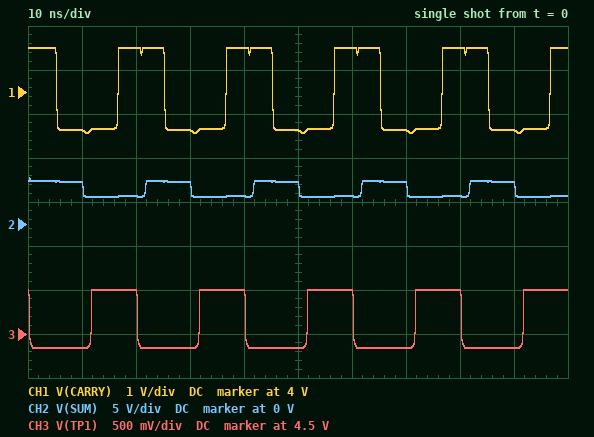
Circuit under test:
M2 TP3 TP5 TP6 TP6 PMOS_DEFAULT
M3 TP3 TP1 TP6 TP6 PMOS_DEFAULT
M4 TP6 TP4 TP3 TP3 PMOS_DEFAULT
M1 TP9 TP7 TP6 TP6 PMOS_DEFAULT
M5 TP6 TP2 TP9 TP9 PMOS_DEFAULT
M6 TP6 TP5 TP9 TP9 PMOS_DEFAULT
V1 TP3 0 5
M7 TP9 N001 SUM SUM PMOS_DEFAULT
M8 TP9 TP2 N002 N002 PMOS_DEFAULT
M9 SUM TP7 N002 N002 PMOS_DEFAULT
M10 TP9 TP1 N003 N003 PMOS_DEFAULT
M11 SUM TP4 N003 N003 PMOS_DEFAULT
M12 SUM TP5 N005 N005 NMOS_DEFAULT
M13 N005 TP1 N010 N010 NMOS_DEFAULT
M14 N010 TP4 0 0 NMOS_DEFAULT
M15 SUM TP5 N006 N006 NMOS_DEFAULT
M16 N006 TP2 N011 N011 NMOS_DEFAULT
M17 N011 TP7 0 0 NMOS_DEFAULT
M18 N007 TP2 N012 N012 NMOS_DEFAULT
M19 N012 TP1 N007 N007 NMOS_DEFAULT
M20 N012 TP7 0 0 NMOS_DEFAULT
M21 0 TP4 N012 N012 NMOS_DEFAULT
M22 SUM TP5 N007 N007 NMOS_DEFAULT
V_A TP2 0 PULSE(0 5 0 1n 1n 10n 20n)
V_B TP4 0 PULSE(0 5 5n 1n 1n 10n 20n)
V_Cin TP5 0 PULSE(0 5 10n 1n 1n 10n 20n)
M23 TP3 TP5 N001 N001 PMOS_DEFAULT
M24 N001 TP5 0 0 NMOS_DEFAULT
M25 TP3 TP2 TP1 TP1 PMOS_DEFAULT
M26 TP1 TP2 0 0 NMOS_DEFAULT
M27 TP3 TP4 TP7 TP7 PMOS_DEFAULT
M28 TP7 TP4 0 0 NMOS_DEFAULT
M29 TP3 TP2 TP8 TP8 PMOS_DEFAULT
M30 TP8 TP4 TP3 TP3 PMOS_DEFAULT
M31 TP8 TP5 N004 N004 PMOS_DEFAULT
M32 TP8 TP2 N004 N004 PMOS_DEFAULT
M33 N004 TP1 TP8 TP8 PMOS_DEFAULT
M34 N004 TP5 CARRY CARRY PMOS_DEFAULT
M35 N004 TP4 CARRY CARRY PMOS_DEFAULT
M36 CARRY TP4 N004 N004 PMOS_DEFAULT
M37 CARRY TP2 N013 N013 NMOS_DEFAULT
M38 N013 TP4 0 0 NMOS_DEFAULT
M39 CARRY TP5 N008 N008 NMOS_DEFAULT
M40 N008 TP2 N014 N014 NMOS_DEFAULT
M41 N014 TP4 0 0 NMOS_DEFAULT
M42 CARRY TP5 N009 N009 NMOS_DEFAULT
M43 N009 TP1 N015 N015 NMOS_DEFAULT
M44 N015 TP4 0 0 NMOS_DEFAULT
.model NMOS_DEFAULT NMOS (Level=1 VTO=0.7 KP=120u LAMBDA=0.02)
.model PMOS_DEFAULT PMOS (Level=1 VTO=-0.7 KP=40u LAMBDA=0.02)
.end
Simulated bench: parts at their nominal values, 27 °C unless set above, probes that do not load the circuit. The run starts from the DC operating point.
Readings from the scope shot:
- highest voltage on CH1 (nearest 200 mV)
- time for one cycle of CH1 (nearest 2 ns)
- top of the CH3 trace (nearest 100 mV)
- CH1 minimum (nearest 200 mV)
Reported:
5.0 V
20 ns
5.0 V
3.0 V
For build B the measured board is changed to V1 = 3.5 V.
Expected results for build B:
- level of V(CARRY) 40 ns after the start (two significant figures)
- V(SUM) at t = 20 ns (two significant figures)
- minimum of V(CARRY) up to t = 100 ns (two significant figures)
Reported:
3.5 V
1.7 V
1.6 V
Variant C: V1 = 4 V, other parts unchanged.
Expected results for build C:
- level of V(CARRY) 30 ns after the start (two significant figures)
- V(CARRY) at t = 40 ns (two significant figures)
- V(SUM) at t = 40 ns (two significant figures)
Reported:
2.1 V
4.0 V
2.2 V
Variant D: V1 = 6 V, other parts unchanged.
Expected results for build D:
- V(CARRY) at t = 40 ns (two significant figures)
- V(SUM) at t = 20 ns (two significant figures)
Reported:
6.0 V
4.1 V
